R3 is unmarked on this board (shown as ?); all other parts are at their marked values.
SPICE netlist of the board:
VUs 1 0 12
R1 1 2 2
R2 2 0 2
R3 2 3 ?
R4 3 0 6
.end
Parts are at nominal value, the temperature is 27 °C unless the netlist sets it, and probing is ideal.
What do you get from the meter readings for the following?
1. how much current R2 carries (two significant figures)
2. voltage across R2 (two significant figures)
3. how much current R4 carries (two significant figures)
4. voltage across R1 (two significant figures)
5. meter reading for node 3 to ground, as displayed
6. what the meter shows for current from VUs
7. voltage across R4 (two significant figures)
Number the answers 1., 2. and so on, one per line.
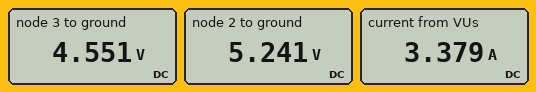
1. 2.6 A
2. 5.2 V
3. 760 mA
4. 6.8 V
5. 4.551 V
6. 3.379 A
7. 4.6 V
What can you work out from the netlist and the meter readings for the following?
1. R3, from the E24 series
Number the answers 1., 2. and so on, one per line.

1. 0.91 Ω
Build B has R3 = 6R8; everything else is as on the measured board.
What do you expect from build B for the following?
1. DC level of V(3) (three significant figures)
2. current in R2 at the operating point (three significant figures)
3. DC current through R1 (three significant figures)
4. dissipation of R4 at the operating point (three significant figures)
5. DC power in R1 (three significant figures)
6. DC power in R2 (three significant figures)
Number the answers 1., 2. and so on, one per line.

1. 2.61 V
2. 2.78 A
3. 3.22 A
4. 1.13 W
5. 20.7 W
6. 15.5 W
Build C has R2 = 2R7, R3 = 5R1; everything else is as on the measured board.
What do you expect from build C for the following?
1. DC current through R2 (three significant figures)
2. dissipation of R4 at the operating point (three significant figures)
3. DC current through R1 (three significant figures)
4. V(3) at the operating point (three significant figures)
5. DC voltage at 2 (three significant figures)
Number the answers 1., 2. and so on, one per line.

1. 2.31 A
2. 1.90 W
3. 2.88 A
4. 3.38 V
5. 6.25 V
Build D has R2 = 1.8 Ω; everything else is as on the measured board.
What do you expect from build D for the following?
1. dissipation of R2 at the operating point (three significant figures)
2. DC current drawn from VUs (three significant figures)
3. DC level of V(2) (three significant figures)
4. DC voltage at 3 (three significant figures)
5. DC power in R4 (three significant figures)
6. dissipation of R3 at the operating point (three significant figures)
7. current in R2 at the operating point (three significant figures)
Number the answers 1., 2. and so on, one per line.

1. 13.9 W
2. 3.50 A
3. 5.00 V
4. 4.34 V
5. 3.14 W
6. 476 mW
7. 2.78 A
